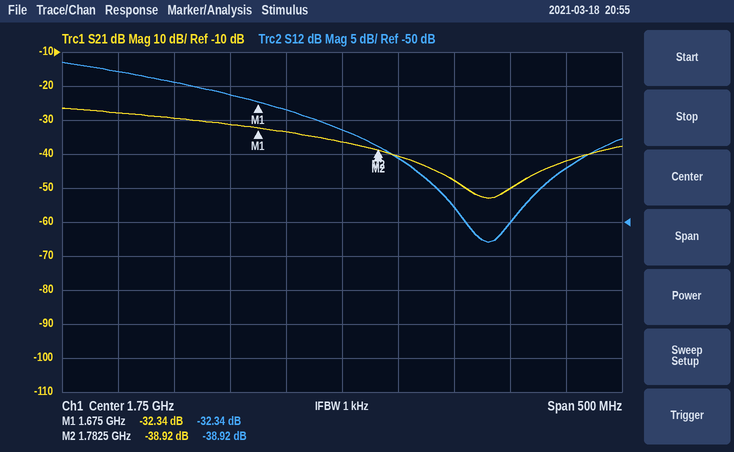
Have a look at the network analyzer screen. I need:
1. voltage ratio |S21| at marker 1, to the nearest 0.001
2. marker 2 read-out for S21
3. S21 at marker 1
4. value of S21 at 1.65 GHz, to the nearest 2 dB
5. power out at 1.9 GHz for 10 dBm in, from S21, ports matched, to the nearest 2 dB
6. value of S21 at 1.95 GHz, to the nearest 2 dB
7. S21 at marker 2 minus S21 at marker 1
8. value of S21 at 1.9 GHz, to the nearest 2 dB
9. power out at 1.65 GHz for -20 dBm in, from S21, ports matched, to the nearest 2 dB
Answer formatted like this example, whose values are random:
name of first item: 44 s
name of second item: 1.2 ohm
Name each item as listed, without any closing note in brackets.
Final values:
voltage ratio |S21| at marker 1, to the nearest 0.001: 0.024
marker 2 read-out for S21: -38.92 dB
S21 at marker 1: -32.34 dB
value of S21 at 1.65 GHz, to the nearest 2 dB: -32 dB
power out at 1.9 GHz for 10 dBm in, from S21, ports matched, to the nearest 2 dB: -40 dBm
value of S21 at 1.95 GHz, to the nearest 2 dB: -42 dB
S21 at marker 2 minus S21 at marker 1: -6.58 dB
value of S21 at 1.9 GHz, to the nearest 2 dB: -50 dB
power out at 1.65 GHz for -20 dBm in, from S21, ports matched, to the nearest 2 dB: -52 dBm
